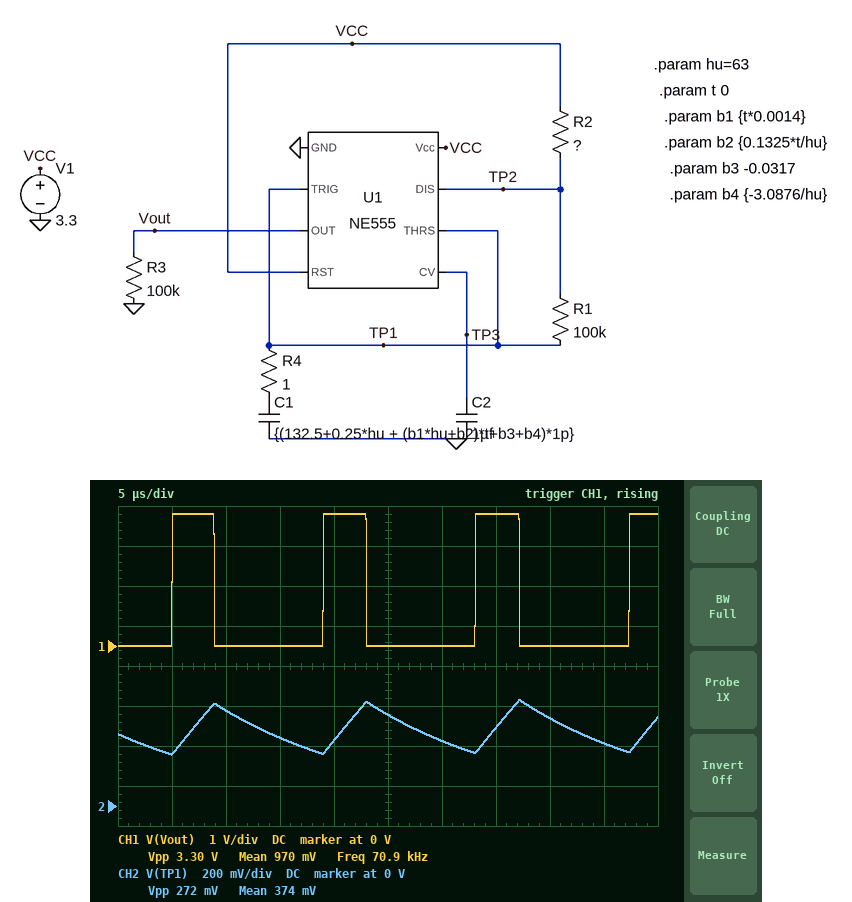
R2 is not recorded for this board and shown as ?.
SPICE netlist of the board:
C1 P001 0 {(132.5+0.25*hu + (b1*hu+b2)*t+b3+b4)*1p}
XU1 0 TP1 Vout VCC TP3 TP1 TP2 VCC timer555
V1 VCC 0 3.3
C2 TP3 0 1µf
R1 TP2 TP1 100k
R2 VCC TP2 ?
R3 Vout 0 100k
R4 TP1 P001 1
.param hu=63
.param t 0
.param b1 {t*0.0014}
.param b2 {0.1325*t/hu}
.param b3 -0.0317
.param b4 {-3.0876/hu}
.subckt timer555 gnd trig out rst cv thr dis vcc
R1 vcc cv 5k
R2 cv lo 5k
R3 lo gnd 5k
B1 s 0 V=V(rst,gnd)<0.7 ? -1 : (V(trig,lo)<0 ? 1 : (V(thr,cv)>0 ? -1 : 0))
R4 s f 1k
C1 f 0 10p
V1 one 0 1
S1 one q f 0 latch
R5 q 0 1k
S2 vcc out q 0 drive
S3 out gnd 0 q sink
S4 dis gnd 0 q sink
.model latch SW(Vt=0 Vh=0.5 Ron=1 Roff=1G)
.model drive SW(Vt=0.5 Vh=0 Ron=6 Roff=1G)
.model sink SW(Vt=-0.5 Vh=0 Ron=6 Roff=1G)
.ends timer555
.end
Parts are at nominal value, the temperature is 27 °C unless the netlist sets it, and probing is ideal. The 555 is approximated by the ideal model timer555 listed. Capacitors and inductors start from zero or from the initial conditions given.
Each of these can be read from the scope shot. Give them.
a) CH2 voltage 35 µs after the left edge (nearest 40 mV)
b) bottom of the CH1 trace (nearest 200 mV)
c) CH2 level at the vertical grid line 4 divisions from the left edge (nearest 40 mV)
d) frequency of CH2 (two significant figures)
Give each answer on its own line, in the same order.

400 mV
0 V
320 mV
71 kHz
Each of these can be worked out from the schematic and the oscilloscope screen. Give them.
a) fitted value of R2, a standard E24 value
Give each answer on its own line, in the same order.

200 kΩ
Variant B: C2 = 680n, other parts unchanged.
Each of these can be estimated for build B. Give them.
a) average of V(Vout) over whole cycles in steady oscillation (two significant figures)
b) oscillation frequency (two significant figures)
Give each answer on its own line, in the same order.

1.2 V
62 kHz
